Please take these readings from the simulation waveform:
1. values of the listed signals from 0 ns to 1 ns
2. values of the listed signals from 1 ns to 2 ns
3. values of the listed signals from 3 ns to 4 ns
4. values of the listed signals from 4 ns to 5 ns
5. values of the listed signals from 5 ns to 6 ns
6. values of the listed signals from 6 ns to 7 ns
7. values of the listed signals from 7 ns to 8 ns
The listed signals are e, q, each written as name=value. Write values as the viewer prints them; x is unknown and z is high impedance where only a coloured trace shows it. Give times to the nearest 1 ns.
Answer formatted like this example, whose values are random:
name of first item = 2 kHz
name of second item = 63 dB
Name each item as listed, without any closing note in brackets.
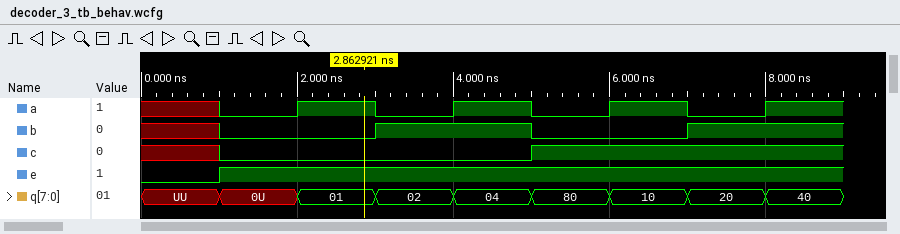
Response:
values of the listed signals from 0 ns to 1 ns = e=0, q=UU
values of the listed signals from 1 ns to 2 ns = e=1, q=0U
values of the listed signals from 3 ns to 4 ns = e=1, q=02
values of the listed signals from 4 ns to 5 ns = e=1, q=04
values of the listed signals from 5 ns to 6 ns = e=1, q=80
values of the listed signals from 6 ns to 7 ns = e=1, q=10
values of the listed signals from 7 ns to 8 ns = e=1, q=20
